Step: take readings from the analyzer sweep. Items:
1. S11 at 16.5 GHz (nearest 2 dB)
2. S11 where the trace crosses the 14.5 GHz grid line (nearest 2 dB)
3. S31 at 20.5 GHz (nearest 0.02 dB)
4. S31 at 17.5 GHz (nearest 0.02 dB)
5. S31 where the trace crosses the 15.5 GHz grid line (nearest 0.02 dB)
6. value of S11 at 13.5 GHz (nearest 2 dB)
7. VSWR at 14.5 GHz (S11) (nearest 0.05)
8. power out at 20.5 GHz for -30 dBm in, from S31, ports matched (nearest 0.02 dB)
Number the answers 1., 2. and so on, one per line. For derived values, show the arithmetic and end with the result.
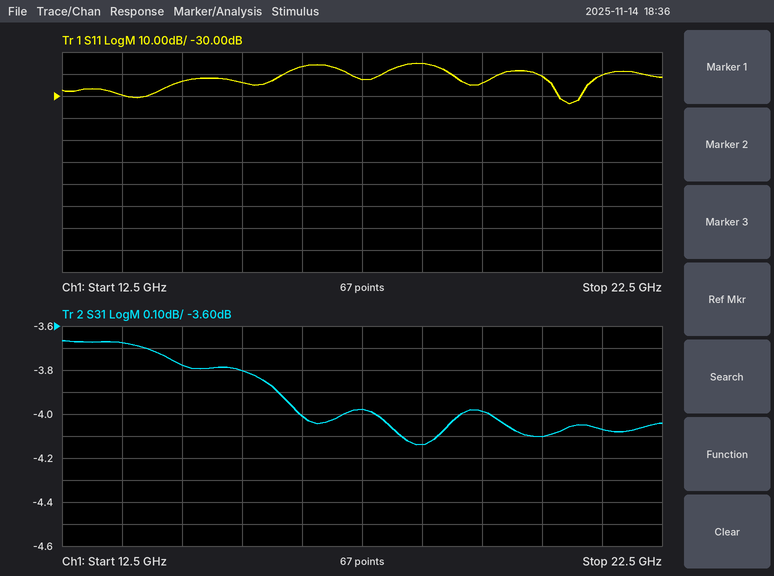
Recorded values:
1. -16 dB
2. -24 dB
3. -4.10 dB
4. -3.98 dB
5. -3.80 dB
6. -30 dB
7. |Γ| = 10^(-24/20) = 0.0631; VSWR = (1 + 0.0631)/(1 − 0.0631) ≈ 1.13, so 1.15 to the nearest 0.05
8. -30 dBm + (-4.10 dB) = -34.10 dBm
